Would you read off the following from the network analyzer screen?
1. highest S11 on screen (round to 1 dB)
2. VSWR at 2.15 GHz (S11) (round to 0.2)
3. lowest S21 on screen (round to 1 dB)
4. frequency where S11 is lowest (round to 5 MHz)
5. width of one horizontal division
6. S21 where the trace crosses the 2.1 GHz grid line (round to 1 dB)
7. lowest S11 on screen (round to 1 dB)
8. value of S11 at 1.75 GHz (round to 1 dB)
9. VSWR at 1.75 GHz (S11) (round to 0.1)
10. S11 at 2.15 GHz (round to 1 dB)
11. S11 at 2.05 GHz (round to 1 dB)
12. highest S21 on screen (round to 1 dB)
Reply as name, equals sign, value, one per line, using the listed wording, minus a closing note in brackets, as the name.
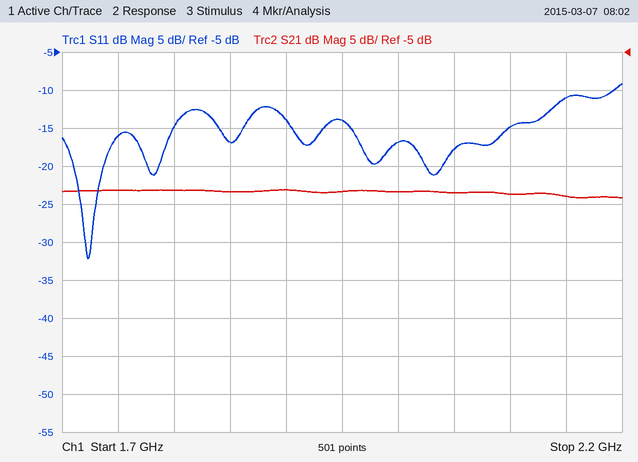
highest S11 on screen = -9 dB
VSWR at 2.15 GHz (S11) = 1.8
lowest S21 on screen = -24 dB
frequency where S11 is lowest = 1.725 GHz
width of one horizontal division = 50 MHz
S21 where the trace crosses the 2.1 GHz grid line = -24 dB
lowest S11 on screen = -32 dB
value of S11 at 1.75 GHz = -16 dB
VSWR at 1.75 GHz (S11) = 1.4
S11 at 2.15 GHz = -11 dB
S11 at 2.05 GHz = -18 dB
highest S21 on screen = -23 dB
